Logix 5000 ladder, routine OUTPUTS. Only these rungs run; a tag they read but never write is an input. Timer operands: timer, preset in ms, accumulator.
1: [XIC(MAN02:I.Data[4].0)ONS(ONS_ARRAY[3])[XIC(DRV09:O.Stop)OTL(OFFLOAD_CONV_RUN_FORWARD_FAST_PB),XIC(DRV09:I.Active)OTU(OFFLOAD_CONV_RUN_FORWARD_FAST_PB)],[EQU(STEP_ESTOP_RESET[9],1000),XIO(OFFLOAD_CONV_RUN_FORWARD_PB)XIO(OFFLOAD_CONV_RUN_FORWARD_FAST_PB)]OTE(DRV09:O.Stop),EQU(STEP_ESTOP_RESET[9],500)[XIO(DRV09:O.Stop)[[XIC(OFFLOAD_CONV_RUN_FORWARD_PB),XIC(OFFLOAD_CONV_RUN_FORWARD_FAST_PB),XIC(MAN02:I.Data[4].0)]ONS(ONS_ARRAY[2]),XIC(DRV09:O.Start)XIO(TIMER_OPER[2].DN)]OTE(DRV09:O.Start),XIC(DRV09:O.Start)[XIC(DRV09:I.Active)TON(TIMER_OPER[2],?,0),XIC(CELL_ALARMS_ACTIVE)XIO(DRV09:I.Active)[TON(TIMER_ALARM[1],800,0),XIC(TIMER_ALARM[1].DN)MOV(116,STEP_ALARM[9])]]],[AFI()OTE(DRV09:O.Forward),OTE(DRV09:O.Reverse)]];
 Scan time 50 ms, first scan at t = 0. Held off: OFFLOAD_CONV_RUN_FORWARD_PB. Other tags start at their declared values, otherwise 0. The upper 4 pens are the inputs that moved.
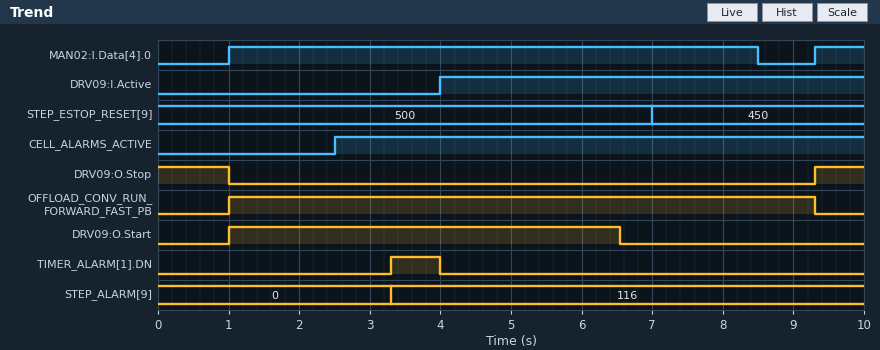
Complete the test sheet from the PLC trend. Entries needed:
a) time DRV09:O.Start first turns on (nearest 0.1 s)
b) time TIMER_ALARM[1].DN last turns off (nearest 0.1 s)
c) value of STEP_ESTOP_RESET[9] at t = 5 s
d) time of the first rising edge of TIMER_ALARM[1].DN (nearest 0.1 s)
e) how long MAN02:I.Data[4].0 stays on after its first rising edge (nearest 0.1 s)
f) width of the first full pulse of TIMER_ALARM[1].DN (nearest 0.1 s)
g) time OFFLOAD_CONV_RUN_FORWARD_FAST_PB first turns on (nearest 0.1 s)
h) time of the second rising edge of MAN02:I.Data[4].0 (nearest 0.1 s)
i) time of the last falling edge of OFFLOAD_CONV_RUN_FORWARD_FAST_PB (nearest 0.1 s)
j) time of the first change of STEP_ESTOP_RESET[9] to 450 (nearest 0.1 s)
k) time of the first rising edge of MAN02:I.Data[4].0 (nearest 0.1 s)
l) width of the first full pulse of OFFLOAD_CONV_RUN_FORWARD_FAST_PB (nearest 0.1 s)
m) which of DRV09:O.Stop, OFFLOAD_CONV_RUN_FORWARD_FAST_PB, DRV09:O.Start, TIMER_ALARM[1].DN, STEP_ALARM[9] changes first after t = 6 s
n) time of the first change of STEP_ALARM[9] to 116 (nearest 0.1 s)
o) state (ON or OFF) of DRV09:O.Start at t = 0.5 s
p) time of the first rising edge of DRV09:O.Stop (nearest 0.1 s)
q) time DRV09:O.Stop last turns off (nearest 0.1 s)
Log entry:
1.0 s
4.0 s
500
3.3 s
7.5 s
0.7 s
1.0 s
9.3 s
9.3 s
7.0 s
1.0 s
8.3 s
DRV09:O.Start
3.3 s
OFF
9.3 s
1.0 s
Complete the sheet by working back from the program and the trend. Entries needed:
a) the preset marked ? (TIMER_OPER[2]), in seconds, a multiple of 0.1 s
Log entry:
2.5 s
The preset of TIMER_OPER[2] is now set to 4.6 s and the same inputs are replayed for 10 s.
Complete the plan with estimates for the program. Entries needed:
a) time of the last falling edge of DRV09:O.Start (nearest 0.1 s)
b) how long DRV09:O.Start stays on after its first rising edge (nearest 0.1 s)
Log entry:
7.0 s
6.0 s
